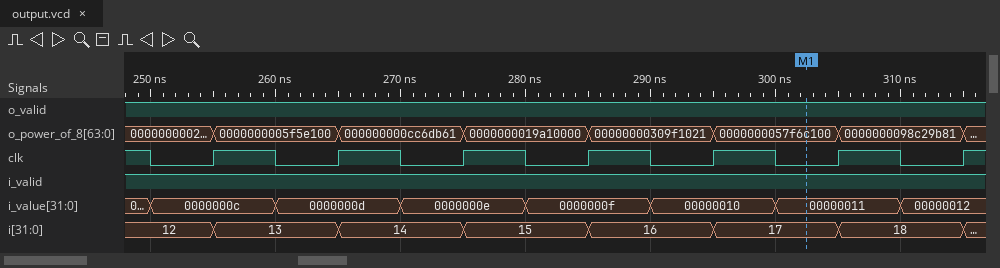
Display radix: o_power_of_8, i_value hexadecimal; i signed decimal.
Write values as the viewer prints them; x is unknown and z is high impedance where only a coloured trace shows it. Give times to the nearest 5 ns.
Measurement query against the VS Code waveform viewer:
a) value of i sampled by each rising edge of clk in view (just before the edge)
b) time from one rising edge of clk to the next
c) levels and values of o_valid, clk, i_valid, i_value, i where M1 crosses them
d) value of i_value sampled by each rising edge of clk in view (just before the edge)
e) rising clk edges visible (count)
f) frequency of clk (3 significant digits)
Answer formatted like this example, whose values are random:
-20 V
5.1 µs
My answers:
12, 13, 14, 15, 16, 17, 18
10 ns
o_valid=1, clk=0, i_valid=1, i_value=00000011, i=17
0000000c, 0000000d, 0000000e, 0000000f, 00000010, 00000011, 00000012
7
100 MHz
